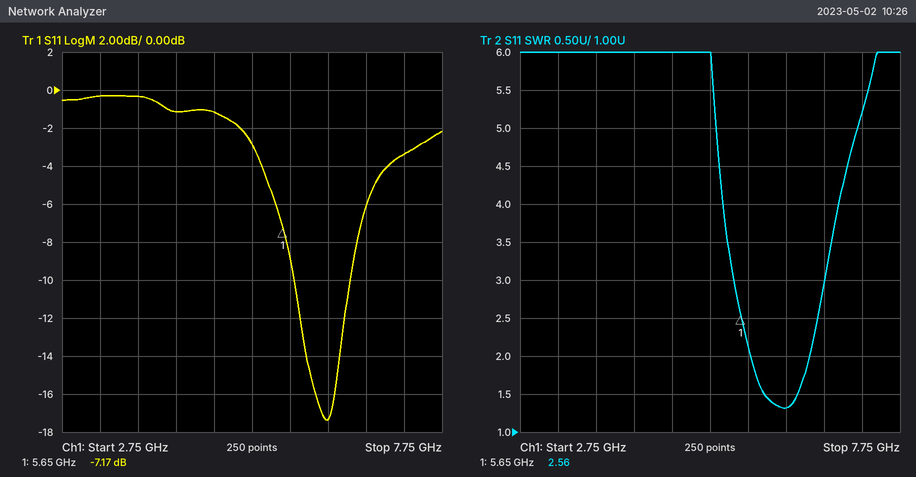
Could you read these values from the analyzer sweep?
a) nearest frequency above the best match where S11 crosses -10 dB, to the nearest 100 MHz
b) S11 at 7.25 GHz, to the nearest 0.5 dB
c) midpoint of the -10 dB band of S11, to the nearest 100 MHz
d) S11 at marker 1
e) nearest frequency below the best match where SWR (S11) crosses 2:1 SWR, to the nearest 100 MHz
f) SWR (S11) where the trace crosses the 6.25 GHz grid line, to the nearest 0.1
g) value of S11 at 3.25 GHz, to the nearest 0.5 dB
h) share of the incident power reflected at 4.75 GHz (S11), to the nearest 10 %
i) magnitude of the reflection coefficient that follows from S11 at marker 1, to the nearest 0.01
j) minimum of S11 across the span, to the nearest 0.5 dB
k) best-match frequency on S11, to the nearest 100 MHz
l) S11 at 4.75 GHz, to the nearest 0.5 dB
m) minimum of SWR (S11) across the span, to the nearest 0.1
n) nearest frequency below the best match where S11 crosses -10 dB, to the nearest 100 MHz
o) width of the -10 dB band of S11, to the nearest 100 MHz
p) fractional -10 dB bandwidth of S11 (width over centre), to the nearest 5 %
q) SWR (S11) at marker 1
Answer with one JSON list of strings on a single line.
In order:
["6.5 GHz", "-3.5 dB", "6.2 GHz", "-7.17 dB", "5.8 GHz", "1.3", "-0.5 dB", "80 %", "0.44", "-17.5 dB", "6.2 GHz", "-1.0 dB", "1.3", "5.8 GHz", "700 MHz", "10 %", "2.56"]
